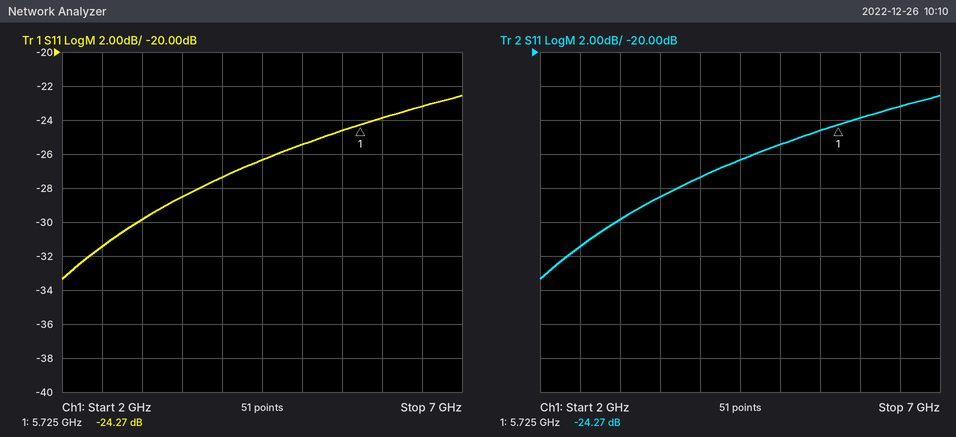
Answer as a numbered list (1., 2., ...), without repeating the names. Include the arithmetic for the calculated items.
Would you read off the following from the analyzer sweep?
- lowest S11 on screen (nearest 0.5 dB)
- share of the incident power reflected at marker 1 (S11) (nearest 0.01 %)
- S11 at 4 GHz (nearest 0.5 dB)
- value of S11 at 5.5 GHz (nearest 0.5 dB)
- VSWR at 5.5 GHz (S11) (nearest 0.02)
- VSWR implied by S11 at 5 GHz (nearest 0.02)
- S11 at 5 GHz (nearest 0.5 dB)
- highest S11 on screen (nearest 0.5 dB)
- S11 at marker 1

1. -33.5 dB
2. 10^(-24.27/10) ≈ 0.37 %
3. -27.5 dB
4. -24.5 dB
5. |Γ| = 10^(-24.5/20) = 0.0596; VSWR = (1 + 0.0596)/(1 − 0.0596) ≈ 1.13, so 1.12 to the nearest 0.02
6. |Γ| = 10^(-25.5/20) = 0.0531; VSWR = (1 + 0.0531)/(1 − 0.0531) ≈ 1.11, so 1.12 to the nearest 0.02
7. -25.5 dB
8. -22.5 dB
9. -24.27 dB
